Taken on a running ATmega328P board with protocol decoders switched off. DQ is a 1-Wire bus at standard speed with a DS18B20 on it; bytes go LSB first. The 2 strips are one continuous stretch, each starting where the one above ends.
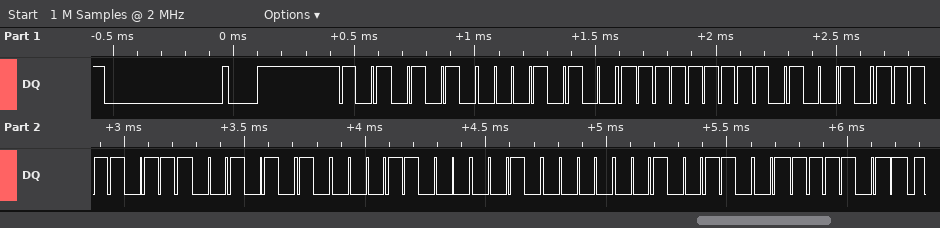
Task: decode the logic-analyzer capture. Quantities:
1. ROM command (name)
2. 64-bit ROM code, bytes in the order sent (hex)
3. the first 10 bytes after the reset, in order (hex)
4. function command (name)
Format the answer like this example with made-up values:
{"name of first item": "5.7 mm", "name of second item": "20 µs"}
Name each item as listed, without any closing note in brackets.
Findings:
{"ROM command": "Match ROM", "64-bit ROM code, bytes in the order sent": "28 FF A5 EF 54 18 04 64", "the first 10 bytes after the reset, in order": "55 28 FF A5 EF 54 18 04 64 BE", "function command": "Read Scratchpad"}
